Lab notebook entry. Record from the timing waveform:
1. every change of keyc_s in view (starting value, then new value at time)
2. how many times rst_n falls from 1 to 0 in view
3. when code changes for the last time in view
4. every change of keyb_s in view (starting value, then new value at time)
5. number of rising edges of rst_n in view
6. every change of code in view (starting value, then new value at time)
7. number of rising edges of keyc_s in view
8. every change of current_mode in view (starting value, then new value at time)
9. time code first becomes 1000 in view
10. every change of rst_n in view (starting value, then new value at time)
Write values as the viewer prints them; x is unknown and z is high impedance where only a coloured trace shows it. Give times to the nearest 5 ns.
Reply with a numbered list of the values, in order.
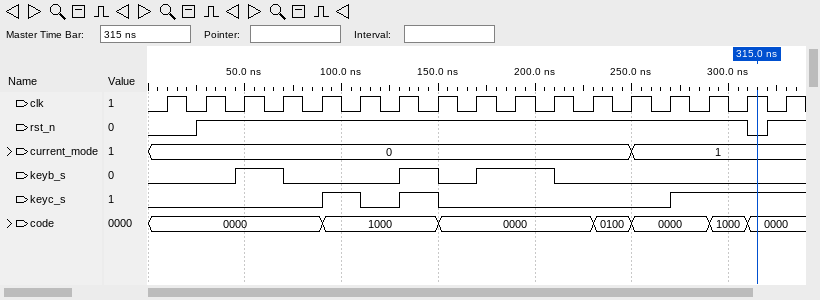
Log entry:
1. 0, 1 at 90 ns, 0 at 110 ns, 1 at 130 ns, 0 at 150 ns, 1 at 270 ns
2. 1
3. 310 ns
4. 0, 1 at 45 ns, 0 at 70 ns, 1 at 130 ns, 0 at 150 ns, 1 at 170 ns, 0 at 210 ns
5. 2
6. 0000, 1000 at 90 ns, 0000 at 150 ns, 0100 at 230 ns, 0000 at 250 ns, 1000 at 290 ns, 0000 at 310 ns
7. 3
8. 0, 1 at 250 ns
9. 90 ns
10. 0, 1 at 25 ns, 0 at 310 ns, 1 at 320 ns
